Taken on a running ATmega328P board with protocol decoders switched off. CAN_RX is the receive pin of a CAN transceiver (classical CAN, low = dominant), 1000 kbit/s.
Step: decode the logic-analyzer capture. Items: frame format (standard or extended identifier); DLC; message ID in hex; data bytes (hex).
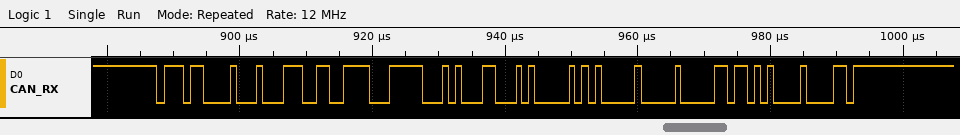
standard
8
0x761
E6 78 F9 46 28 14 00 05
